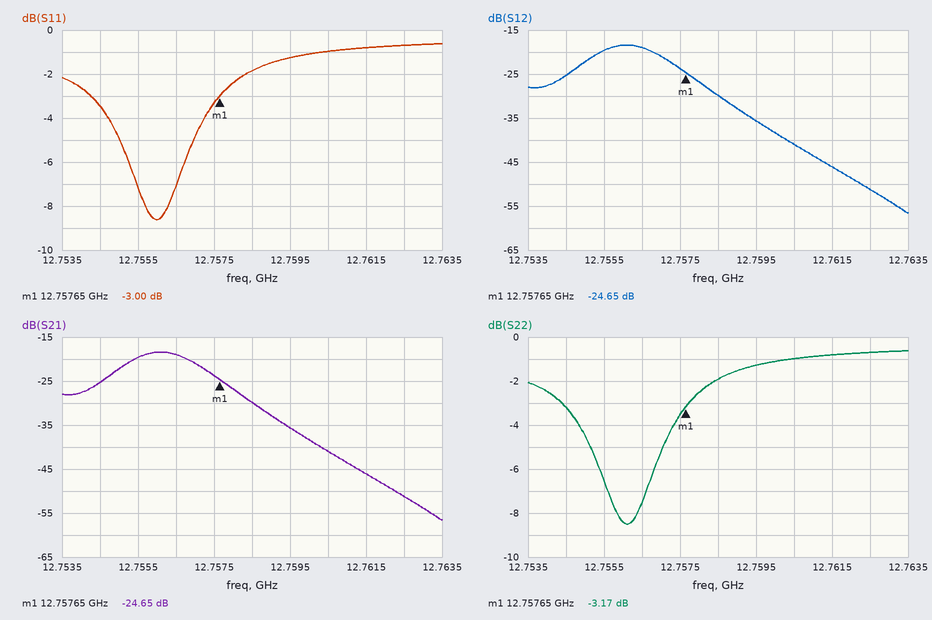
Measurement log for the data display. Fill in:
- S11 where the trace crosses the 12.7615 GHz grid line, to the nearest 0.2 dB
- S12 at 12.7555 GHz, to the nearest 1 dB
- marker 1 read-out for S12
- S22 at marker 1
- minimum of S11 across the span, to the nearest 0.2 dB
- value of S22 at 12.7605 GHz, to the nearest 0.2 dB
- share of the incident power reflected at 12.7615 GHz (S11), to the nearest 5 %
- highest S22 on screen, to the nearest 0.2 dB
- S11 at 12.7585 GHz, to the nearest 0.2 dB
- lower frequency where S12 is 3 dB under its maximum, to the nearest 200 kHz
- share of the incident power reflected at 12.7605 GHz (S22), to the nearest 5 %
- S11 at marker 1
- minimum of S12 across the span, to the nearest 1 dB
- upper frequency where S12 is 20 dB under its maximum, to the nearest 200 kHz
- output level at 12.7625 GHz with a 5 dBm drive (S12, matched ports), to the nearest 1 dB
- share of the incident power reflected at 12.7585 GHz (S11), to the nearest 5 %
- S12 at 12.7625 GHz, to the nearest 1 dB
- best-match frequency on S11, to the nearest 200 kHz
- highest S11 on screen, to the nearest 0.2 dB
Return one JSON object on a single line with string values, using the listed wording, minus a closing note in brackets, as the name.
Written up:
{"S11 where the trace crosses the 12.7615 GHz grid line, to the nearest 0.2 dB": "-0.8 dB", "S12 at 12.7555 GHz, to the nearest 1 dB": "-20 dB", "marker 1 read-out for S12": "-24.65 dB", "S22 at marker 1": "-3.17 dB", "minimum of S11 across the span, to the nearest 0.2 dB": "-8.6 dB", "value of S22 at 12.7605 GHz, to the nearest 0.2 dB": "-1.0 dB", "share of the incident power reflected at 12.7615 GHz (S11), to the nearest 5 %": "85 %", "highest S22 on screen, to the nearest 0.2 dB": "-0.6 dB", "S11 at 12.7585 GHz, to the nearest 0.2 dB": "-1.8 dB", "lower frequency where S12 is 3 dB under its maximum, to the nearest 200 kHz": "12.7552 GHz", "share of the incident power reflected at 12.7605 GHz (S22), to the nearest 5 %": "80 %", "S11 at marker 1": "-3.00 dB", "minimum of S12 across the span, to the nearest 1 dB": "-57 dB", "upper frequency where S12 is 20 dB under its maximum, to the nearest 200 kHz": "12.7600 GHz", "output level at 12.7625 GHz with a 5 dBm drive (S12, matched ports), to the nearest 1 dB": "-46 dBm", "share of the incident power reflected at 12.7585 GHz (S11), to the nearest 5 %": "65 %", "S12 at 12.7625 GHz, to the nearest 1 dB": "-51 dB", "best-match frequency on S11, to the nearest 200 kHz": "12.7560 GHz", "highest S11 on screen, to the nearest 0.2 dB": "-0.6 dB"}
